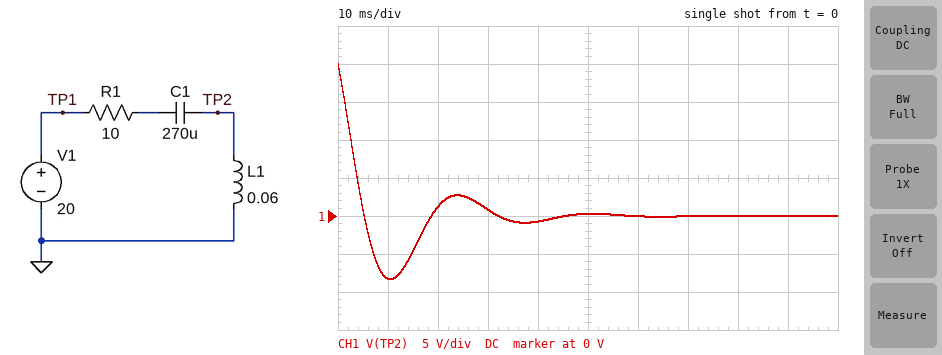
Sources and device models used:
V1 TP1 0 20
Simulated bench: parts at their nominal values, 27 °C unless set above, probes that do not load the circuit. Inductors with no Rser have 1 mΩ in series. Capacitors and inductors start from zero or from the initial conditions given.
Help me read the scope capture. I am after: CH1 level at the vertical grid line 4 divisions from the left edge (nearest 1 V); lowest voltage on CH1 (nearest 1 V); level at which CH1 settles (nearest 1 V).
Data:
-1 V
-8 V
0 V
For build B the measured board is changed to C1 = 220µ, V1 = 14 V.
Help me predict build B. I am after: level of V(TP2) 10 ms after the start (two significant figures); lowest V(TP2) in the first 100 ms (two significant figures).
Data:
-6.2 V
-6.3 V
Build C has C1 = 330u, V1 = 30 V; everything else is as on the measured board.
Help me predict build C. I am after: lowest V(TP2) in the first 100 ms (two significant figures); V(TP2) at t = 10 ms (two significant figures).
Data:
-12 V
-11 V
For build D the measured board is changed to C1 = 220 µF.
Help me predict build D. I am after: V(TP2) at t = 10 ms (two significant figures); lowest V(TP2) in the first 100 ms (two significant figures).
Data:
-8.9 V
-9.0 V
